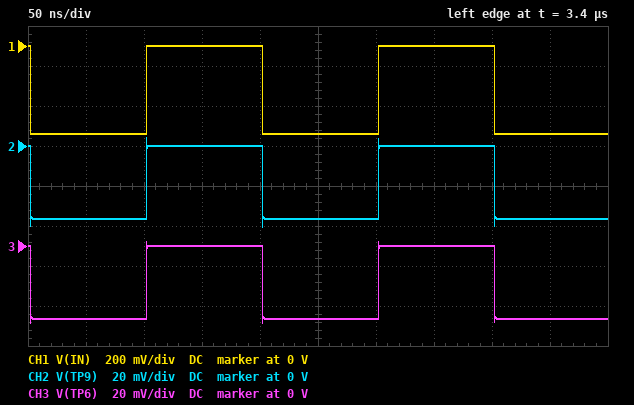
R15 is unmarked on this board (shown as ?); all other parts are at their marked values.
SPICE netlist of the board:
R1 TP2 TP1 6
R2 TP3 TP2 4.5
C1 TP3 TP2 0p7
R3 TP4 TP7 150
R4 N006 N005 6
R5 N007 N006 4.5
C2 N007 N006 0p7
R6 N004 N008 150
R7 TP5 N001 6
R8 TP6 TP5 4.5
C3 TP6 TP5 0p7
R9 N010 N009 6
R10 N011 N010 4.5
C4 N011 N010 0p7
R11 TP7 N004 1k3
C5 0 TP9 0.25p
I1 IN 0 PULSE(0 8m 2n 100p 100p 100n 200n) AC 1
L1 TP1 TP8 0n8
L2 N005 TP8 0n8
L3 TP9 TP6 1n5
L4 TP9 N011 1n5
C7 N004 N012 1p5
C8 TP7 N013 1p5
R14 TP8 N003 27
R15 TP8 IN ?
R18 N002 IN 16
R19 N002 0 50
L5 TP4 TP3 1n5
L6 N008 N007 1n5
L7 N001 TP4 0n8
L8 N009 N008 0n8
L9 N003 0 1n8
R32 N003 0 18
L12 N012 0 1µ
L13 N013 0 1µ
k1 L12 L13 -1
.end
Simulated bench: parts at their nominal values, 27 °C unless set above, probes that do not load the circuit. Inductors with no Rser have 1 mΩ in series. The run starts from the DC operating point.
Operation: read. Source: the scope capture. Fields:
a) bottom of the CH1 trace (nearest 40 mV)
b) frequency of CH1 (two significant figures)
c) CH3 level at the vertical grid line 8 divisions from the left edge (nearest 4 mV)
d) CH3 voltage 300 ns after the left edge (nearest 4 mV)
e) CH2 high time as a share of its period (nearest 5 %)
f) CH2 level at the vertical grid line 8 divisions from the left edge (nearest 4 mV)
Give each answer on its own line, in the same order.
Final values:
-440 mV
5.0 MHz
0 V
-36 mV
50 %
0 V
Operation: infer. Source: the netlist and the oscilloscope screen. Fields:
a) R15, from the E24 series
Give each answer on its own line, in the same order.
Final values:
300 Ω
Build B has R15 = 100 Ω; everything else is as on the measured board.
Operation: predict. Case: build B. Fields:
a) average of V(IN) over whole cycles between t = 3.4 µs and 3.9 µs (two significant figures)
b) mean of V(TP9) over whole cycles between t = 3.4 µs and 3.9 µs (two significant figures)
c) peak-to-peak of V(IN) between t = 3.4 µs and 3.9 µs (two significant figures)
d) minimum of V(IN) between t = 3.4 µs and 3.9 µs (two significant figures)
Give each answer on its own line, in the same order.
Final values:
-170 mV
-37 mV
350 mV
-350 mV
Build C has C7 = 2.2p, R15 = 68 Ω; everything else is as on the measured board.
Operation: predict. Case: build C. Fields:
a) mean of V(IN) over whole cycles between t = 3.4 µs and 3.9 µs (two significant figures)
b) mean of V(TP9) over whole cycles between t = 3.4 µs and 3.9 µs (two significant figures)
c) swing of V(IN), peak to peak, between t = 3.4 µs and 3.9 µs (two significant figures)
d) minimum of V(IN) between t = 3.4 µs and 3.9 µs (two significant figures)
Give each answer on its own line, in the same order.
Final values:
-160 mV
-44 mV
310 mV
-310 mV
